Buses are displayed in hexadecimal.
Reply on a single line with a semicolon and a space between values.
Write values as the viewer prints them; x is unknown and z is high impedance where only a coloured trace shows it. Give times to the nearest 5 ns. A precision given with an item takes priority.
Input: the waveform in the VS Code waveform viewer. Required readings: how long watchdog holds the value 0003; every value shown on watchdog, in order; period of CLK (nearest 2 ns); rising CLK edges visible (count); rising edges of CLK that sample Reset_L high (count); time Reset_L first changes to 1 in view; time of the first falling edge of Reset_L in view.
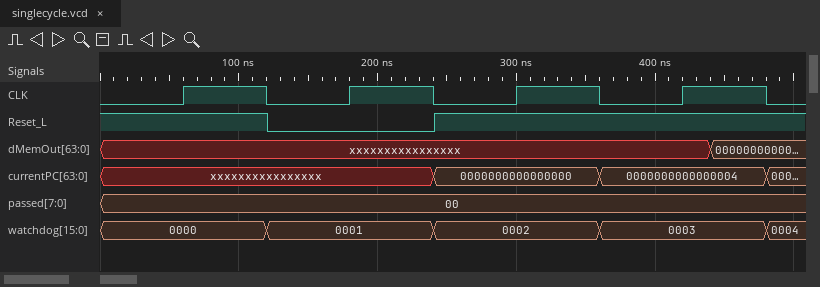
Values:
120 ns; 0000, 0001, 0002, 0003, 0004; 120 ns; 4; 3; 240 ns; 120 ns
